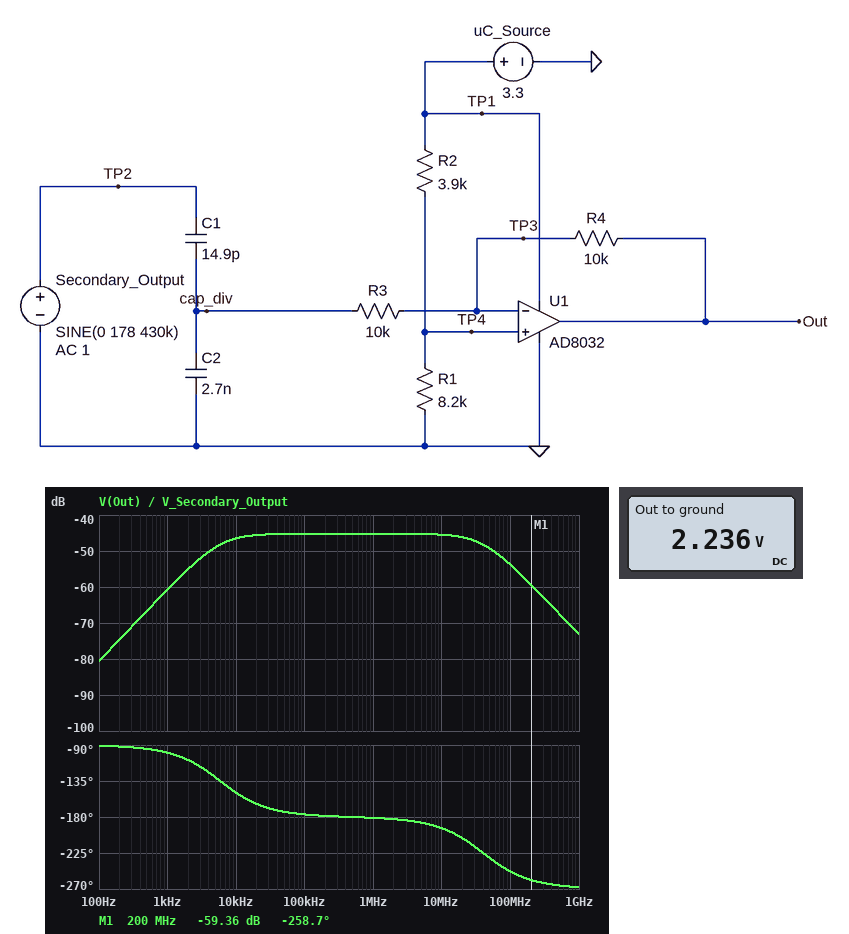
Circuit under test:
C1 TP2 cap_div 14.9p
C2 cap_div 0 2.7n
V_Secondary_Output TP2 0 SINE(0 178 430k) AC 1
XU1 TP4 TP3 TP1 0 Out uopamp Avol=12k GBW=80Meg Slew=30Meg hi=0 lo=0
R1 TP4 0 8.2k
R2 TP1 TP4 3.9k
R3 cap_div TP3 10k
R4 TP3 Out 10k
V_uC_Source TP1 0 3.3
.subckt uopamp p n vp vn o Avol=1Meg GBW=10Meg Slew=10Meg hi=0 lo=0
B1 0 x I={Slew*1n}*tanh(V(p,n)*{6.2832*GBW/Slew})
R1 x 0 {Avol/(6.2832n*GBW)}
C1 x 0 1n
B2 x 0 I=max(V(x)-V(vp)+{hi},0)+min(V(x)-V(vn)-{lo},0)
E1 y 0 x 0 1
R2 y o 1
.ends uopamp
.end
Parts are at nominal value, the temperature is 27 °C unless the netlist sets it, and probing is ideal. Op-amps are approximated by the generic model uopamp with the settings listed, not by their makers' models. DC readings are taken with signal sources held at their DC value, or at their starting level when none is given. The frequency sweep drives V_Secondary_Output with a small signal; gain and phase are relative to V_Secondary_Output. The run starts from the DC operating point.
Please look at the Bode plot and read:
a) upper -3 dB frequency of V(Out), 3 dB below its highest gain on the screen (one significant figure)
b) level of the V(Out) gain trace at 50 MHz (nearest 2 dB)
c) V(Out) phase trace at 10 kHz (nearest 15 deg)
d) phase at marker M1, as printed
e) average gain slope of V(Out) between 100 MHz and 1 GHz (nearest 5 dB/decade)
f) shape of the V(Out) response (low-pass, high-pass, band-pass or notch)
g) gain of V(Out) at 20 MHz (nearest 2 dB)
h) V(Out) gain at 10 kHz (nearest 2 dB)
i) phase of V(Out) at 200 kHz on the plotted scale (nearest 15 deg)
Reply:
40 MHz
-50 dB
-150 deg
-258.7 deg
-20 dB/decade
band-pass
-46 dB
-46 dB
-180 deg
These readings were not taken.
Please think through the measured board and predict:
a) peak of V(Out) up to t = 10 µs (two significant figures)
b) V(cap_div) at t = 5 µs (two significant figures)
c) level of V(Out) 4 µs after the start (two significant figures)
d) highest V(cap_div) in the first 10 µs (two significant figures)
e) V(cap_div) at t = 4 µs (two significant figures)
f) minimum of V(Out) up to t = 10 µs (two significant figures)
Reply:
3.2 V
3.0 V
3.2 V
3.2 V
1.3 V
1.3 V
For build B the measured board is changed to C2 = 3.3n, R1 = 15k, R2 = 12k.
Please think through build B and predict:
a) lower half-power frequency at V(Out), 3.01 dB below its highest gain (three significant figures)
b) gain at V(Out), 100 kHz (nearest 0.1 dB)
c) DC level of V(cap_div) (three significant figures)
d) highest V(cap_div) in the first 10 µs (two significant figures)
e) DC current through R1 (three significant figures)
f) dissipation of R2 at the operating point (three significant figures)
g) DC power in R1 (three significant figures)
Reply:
4.80 kHz
-47.0 dB
1.83 V
2.6 V
122 µA
179 µW
224 µW
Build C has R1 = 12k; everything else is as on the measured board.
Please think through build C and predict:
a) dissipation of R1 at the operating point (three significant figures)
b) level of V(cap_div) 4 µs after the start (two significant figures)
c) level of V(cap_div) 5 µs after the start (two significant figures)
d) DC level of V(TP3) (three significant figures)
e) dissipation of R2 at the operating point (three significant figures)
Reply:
517 µW
1.5 V
3.3 V
2.49 V
168 µW
